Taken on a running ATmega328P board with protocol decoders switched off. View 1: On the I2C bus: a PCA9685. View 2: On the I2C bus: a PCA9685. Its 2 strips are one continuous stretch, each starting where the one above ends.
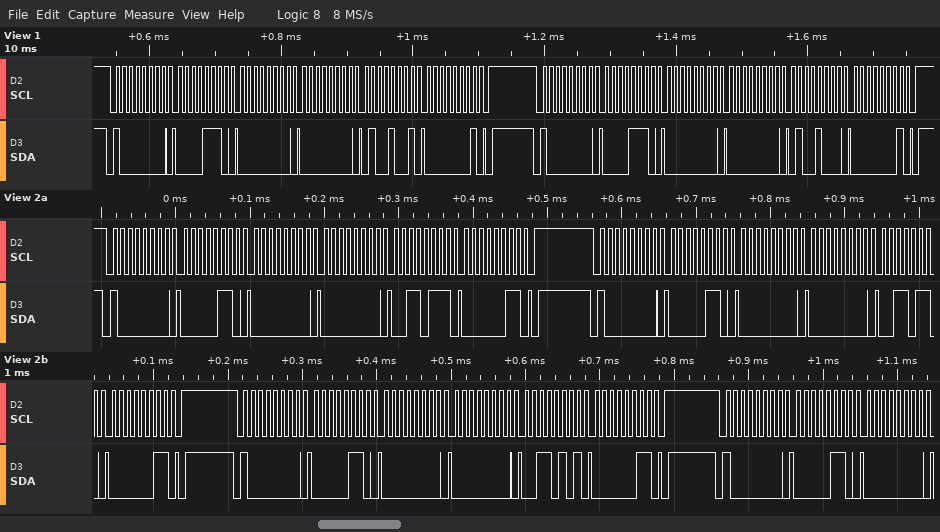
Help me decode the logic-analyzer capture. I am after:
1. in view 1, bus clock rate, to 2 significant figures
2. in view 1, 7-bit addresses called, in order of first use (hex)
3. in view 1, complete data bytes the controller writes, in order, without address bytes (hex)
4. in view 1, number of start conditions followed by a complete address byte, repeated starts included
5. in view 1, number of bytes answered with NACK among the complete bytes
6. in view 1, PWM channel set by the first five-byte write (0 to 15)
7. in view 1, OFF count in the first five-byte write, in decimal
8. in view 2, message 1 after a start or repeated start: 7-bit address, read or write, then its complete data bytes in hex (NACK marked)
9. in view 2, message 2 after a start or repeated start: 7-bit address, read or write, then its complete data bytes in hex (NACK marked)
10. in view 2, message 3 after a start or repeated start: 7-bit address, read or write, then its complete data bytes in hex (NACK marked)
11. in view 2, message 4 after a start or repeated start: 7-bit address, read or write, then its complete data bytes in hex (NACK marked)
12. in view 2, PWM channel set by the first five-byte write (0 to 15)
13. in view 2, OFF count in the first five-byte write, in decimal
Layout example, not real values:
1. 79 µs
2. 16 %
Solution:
1. 100 kHz
2. 0x40
3. 0E 00 00 49 01 0E 00 00 48 01
4. 2
5. 0
6. 2
7. 329
8. 0x40 write: 06 00 00 37 03
9. 0x40 write: 06 00 00 36 03
10. 0x40 write: 06 00 00 35 03
11. 0x40 write: 06 00
12. 0
13. 823
